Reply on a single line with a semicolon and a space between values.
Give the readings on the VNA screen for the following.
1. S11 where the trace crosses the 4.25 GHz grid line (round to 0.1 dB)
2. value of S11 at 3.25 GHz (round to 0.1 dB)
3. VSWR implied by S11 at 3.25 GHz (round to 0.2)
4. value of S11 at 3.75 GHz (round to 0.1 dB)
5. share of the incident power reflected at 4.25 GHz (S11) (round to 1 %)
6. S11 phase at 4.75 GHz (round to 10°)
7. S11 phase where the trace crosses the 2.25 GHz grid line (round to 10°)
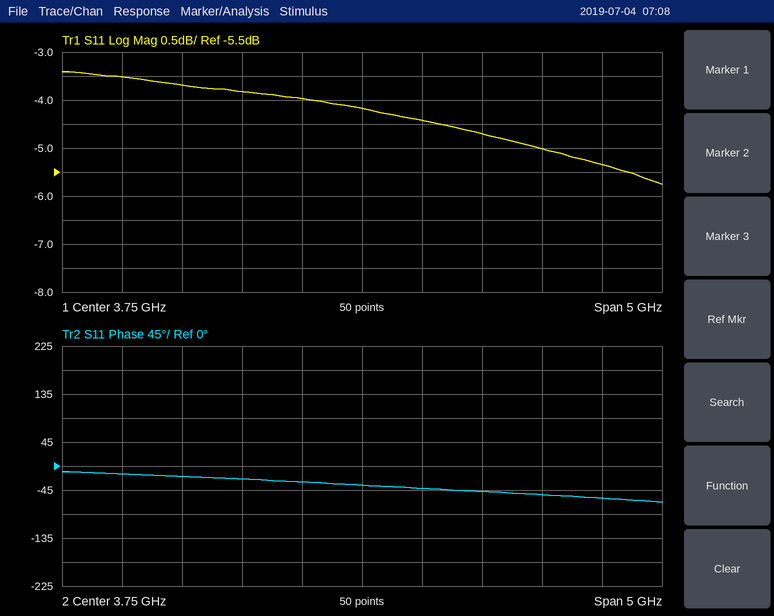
-4.4 dB; -4.0 dB; 4.4; -4.2 dB; 36 %; -50°; -20°
